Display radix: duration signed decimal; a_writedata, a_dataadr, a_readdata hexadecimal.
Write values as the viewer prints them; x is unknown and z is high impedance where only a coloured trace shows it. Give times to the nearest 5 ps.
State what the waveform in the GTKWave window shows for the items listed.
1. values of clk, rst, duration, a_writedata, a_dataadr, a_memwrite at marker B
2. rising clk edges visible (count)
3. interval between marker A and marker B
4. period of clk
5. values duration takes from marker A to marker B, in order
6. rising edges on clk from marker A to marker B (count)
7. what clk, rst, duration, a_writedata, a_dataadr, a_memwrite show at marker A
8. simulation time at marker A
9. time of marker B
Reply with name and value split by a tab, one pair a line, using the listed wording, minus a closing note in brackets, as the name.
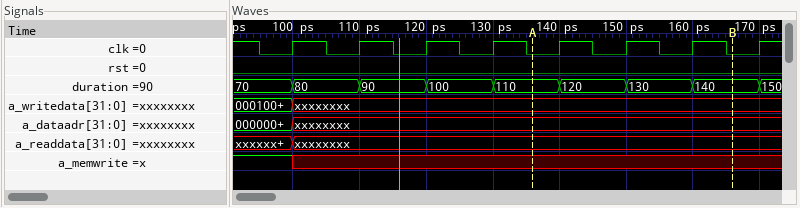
values of clk, rst, duration, a_writedata, a_dataadr, a_memwrite at marker B	clk=0, rst=0, duration=140, a_writedata=xxxxxxxx, a_dataadr=xxxxxxxx, a_memwrite=x
rising clk edges visible	8
interval between marker A and marker B	30 ps
period of clk	10 ps
values duration takes from marker A to marker B, in order	110, 120, 130, 140
rising edges on clk from marker A to marker B	3
what clk, rst, duration, a_writedata, a_dataadr, a_memwrite show at marker A	clk=0, rst=0, duration=110, a_writedata=xxxxxxxx, a_dataadr=xxxxxxxx, a_memwrite=x
simulation time at marker A	135 ps
time of marker B	165 ps
